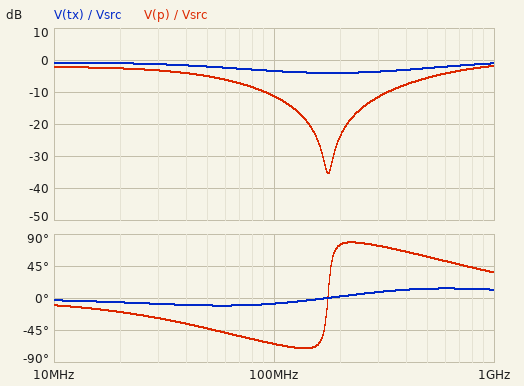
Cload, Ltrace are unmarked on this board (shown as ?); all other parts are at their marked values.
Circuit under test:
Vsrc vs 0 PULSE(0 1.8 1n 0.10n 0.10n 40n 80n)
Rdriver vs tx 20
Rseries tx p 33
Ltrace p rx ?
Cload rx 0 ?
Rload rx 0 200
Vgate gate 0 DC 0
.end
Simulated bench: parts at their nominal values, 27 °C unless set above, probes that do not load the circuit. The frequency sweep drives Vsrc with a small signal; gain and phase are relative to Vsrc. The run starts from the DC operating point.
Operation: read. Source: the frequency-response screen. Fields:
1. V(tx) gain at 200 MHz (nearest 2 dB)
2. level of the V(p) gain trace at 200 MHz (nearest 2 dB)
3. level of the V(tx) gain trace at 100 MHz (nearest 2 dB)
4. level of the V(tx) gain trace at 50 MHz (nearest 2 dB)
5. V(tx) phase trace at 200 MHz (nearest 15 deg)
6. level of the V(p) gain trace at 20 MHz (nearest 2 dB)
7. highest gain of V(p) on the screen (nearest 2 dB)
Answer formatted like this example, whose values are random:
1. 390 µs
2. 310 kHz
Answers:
1. -4 dB
2. -24 dB
3. -4 dB
4. -2 dB
5. 0 deg
6. -2 dB
7. -2 dB
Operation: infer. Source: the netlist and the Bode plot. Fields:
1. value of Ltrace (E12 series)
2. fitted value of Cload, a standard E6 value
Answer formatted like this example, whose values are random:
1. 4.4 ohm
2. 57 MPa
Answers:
1. 12 nH
2. 68 pF
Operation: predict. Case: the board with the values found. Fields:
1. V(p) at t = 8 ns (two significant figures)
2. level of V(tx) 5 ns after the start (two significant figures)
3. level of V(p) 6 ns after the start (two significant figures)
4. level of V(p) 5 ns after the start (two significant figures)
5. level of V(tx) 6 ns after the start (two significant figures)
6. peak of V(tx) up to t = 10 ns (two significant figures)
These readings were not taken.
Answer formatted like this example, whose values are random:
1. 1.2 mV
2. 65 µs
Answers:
1. 1.3 V
2. 1.5 V
3. 1.2 V
4. 1.0 V
5. 1.6 V
6. 1.7 V
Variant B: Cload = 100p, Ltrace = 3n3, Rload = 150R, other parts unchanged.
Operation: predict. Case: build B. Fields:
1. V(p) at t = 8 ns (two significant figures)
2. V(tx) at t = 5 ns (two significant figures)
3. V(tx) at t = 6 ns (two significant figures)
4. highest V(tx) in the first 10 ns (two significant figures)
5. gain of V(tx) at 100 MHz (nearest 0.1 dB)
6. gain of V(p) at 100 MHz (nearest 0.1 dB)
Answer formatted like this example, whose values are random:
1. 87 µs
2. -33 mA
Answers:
1. 1.1 V
2. 1.4 V
3. 1.5 V
4. 1.6 V
5. -3.6 dB
6. -12.2 dB
